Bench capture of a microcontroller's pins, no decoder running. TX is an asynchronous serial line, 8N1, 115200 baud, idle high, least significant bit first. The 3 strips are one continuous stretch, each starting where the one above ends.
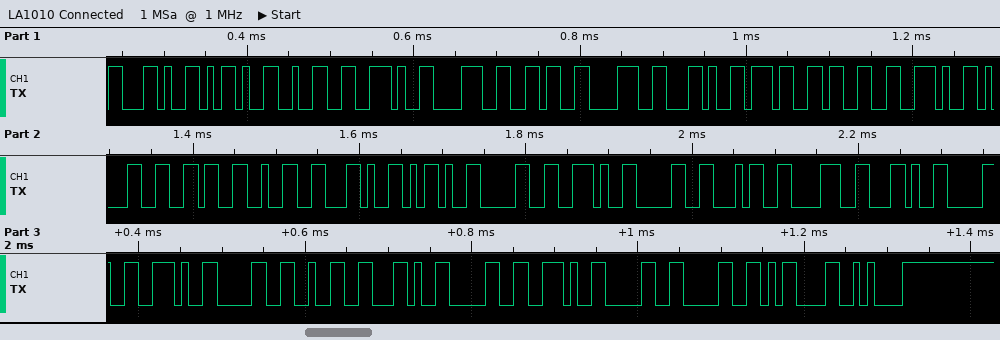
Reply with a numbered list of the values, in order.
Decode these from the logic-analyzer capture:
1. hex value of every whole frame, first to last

1. 2C 2D 32 2E 38 36 38 2C 37 33 2E 31 36 32 2C 2D 30 2E 30 34 38 2C 30 2E 30 32 2C 30 2E 30 30 0D 0A
